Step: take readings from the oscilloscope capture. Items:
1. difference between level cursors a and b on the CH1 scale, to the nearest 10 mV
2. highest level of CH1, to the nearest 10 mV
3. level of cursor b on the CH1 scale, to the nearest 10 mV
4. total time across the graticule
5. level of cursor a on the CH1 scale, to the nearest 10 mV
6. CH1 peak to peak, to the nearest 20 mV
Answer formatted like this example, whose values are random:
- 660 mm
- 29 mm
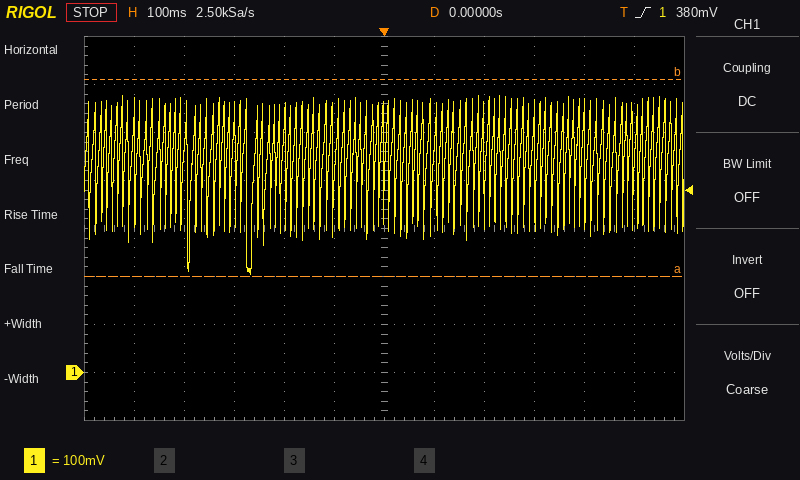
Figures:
- 410 mV
- 580 mV
- 610 mV
- 1.2 s
- 200 mV
- 380 mV
